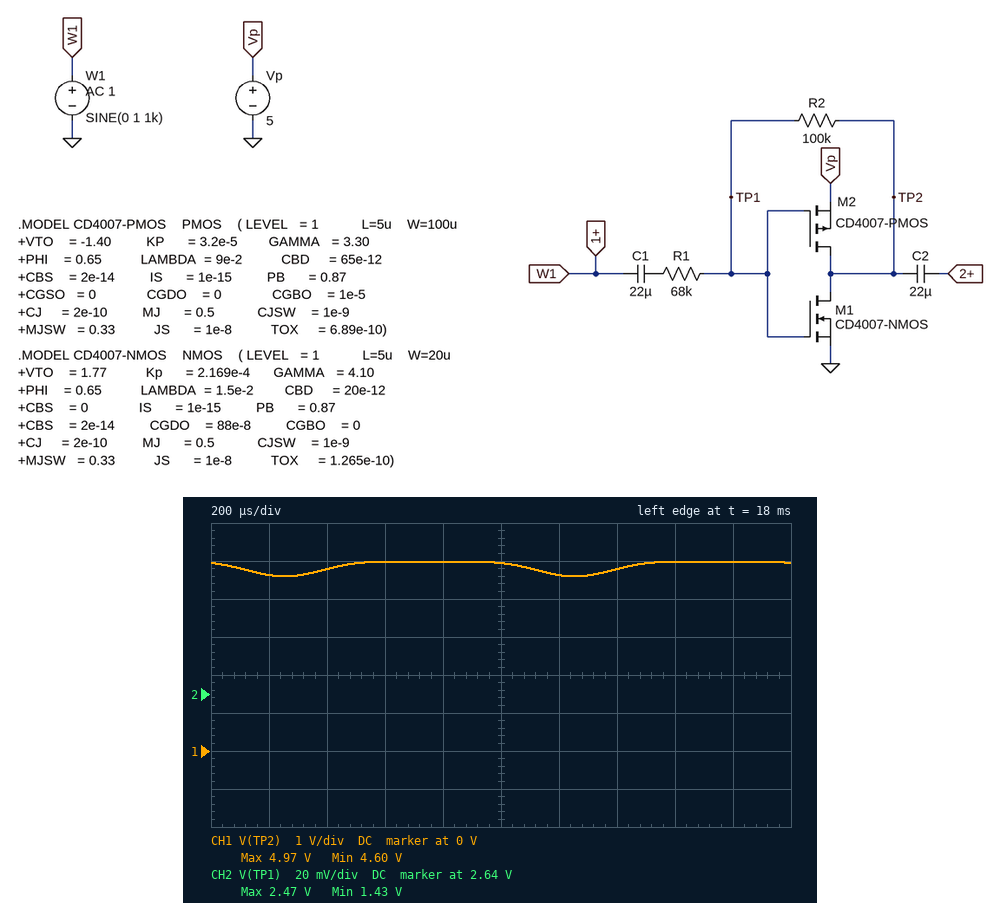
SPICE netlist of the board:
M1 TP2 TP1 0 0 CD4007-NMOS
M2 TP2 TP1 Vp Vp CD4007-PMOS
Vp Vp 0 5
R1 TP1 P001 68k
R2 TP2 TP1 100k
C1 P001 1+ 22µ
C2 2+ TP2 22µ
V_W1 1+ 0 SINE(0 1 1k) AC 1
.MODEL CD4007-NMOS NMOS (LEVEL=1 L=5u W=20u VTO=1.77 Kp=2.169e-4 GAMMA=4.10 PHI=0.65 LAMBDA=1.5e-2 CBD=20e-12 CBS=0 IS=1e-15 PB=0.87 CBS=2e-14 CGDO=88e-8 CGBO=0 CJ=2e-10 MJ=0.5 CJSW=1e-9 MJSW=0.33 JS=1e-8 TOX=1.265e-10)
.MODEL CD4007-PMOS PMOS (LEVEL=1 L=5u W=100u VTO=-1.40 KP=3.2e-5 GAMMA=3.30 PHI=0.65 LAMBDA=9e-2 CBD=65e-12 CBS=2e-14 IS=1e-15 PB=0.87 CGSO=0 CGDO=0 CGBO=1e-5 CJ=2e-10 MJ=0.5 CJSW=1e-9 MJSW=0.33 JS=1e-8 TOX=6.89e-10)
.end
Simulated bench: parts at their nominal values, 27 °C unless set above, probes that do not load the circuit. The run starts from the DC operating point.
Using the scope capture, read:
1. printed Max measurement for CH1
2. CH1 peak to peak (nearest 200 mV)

4.97 V
400 mV
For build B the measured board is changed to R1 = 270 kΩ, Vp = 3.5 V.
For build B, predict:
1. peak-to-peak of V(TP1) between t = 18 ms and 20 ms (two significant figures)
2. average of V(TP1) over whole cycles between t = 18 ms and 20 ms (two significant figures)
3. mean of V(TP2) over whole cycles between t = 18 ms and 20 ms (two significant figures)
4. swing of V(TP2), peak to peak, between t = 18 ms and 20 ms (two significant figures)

32 mV
1.9 V
2.6 V
700 mV
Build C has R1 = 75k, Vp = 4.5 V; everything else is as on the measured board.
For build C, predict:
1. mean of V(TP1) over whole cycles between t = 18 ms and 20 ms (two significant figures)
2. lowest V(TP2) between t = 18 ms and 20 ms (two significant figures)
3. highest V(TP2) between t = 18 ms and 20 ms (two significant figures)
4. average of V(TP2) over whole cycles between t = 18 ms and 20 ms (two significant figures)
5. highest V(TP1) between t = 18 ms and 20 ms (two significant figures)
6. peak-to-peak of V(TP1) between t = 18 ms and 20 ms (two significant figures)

1.9 V
4.1 V
4.5 V
4.4 V
2.3 V
970 mV
